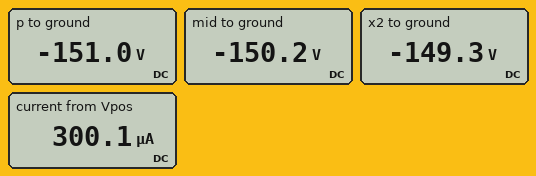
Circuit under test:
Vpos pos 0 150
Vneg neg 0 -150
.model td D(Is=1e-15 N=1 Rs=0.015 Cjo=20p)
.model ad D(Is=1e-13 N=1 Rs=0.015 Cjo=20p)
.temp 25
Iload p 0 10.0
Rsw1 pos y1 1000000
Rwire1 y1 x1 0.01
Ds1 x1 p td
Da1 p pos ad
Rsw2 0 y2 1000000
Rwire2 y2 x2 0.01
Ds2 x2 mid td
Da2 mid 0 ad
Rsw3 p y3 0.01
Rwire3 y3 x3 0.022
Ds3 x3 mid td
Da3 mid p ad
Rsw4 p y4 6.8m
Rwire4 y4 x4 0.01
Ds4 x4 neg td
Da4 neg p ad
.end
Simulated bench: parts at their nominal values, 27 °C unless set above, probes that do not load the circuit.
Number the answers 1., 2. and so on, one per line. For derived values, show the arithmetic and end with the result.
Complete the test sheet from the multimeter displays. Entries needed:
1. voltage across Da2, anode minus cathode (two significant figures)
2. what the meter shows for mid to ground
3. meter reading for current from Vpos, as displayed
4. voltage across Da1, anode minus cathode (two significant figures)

1. -150.2 V = -150 V
2. -150.2 V
3. 300.1 µA
4. -151 V - 150 V = -300 V
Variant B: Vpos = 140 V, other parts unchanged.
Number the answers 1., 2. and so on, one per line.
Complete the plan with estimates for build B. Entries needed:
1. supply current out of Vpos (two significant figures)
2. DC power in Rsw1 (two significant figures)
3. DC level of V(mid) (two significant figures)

1. 290 µA
2. 84 mW
3. -150 V
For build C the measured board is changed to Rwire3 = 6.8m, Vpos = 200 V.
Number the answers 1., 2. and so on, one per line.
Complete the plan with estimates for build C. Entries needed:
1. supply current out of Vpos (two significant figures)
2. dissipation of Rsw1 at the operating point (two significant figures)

1. 350 µA
2. 120 mW
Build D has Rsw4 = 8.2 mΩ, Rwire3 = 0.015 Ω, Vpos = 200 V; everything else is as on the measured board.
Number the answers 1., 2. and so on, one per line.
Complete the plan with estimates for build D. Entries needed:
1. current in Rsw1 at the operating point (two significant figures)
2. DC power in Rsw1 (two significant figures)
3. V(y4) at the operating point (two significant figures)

1. 350 µA
2. 120 mW
3. -150 V
